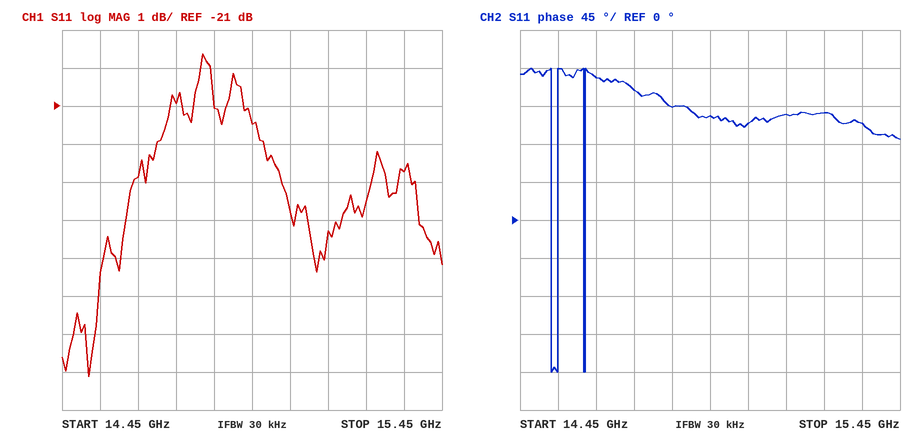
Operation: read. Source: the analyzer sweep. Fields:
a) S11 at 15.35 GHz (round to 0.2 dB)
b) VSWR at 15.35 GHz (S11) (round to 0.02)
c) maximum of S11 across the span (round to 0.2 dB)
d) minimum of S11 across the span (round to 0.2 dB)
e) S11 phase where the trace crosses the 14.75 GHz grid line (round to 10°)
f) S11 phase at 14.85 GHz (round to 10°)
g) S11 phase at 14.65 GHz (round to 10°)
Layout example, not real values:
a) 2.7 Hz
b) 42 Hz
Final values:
a) -22.8 dB
b) 1.16
c) -19.6 dB
d) -28.2 dB
e) 150°
f) 130°
g) 170°
